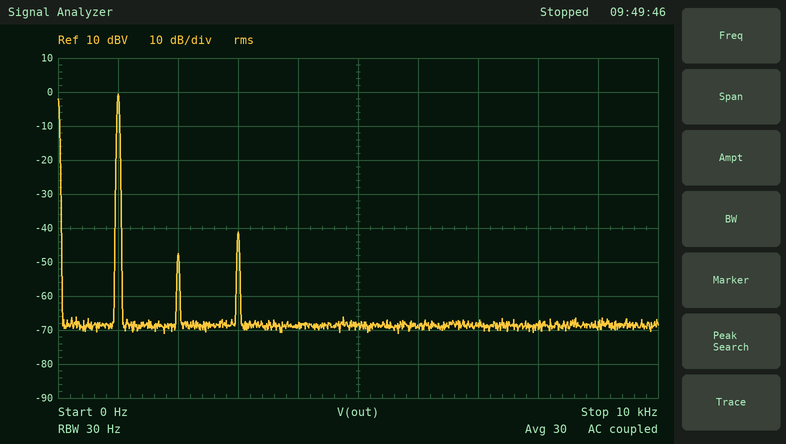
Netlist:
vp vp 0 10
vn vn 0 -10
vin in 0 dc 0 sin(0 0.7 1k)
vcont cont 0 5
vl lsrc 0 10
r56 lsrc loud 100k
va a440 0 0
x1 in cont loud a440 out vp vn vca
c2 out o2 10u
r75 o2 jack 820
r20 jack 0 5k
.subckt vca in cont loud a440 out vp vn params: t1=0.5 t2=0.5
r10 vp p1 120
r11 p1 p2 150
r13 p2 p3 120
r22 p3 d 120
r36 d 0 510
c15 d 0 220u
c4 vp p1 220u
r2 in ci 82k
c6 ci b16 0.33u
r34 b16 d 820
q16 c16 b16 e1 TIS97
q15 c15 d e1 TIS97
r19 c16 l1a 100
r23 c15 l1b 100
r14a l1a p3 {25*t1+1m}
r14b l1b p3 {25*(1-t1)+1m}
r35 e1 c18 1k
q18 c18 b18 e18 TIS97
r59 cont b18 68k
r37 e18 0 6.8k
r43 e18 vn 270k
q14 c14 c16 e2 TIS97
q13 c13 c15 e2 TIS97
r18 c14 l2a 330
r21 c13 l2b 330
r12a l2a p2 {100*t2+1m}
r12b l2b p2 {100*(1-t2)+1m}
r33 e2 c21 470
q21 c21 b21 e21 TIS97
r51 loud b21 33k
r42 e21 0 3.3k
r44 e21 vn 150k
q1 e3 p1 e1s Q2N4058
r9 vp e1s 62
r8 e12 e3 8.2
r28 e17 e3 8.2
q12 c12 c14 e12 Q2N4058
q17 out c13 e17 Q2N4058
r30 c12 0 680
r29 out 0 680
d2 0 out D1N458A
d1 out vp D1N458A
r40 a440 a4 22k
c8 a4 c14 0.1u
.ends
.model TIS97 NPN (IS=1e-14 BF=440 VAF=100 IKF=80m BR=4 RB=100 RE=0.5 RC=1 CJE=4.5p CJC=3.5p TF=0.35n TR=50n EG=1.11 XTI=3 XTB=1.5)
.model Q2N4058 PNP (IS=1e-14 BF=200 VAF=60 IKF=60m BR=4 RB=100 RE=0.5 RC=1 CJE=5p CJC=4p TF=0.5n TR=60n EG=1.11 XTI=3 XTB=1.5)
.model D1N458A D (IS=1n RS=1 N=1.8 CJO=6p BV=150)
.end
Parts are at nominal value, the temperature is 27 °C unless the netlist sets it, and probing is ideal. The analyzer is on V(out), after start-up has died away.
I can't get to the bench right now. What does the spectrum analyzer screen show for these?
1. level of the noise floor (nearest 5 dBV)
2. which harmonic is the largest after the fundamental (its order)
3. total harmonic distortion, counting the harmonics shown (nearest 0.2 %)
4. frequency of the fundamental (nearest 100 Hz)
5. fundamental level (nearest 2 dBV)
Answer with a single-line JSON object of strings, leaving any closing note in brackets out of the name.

{"level of the noise floor": "-70 dBV", "which harmonic is the largest after the fundamental": "3", "total harmonic distortion, counting the harmonics shown": "1.0 %", "frequency of the fundamental": "1.0 kHz", "fundamental level": "0 dBV"}
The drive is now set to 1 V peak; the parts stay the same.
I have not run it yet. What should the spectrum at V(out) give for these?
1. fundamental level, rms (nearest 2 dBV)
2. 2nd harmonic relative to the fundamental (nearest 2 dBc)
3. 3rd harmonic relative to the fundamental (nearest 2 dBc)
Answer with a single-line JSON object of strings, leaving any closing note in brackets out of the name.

{"fundamental level, rms": "2 dBV", "2nd harmonic relative to the fundamental": "-44 dBc", "3rd harmonic relative to the fundamental": "-34 dBc"}
